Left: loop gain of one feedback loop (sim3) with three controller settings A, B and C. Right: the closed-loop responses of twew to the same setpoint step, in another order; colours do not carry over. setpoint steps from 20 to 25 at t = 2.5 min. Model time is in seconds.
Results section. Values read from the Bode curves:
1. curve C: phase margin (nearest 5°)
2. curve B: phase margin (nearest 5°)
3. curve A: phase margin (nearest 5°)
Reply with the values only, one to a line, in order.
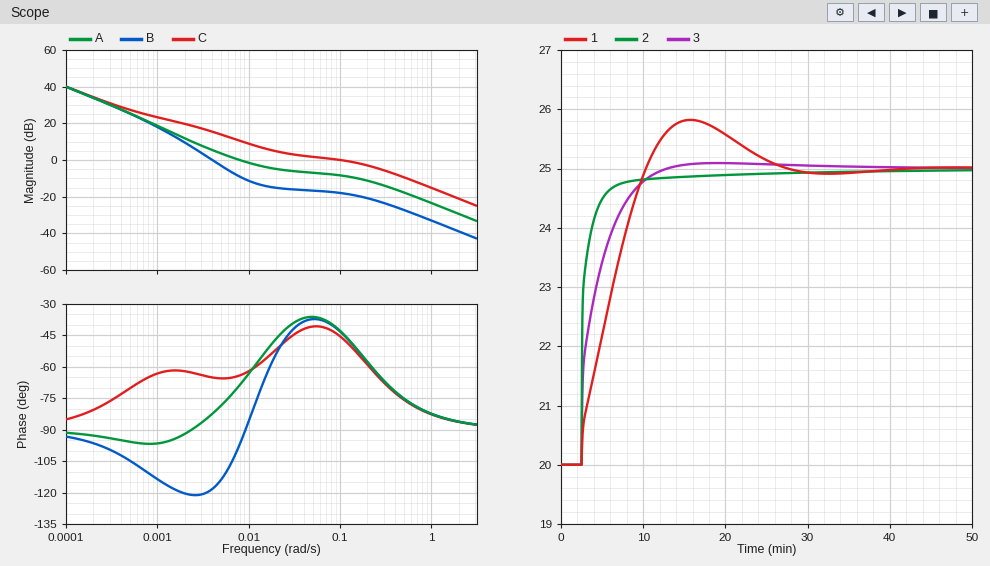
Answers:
135°
60°
110°
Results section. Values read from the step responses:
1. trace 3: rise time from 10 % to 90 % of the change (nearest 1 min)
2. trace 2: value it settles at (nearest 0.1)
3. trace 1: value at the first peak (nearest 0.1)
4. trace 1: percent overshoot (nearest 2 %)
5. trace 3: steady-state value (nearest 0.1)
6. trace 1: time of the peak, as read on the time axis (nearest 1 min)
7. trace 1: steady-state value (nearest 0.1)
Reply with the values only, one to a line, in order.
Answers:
6 min
25.0
25.8
16 %
25.0
16 min
25.0
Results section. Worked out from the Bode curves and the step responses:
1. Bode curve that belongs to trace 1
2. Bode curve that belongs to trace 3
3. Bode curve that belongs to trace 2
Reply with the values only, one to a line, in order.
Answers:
B
A
C
